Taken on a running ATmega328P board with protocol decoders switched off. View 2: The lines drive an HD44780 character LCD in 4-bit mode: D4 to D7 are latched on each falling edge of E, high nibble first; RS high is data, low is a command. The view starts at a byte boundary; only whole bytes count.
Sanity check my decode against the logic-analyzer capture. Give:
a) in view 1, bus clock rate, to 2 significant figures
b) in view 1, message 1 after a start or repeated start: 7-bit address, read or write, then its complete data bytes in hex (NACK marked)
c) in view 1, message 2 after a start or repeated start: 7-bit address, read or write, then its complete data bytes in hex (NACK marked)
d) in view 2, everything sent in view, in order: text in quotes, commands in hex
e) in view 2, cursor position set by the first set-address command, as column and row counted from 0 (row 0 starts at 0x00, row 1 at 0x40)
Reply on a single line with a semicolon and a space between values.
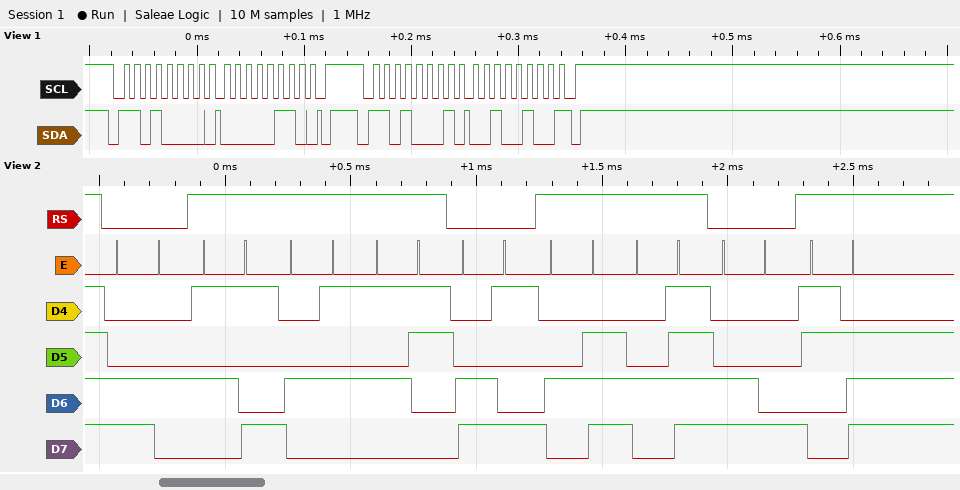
100 kHz; 0x68 write: 06; 0x68 read: 24 NACK; 0xC4 "YES" 0xC9 "NO" 0xC8 ">"; column 4, row 1
